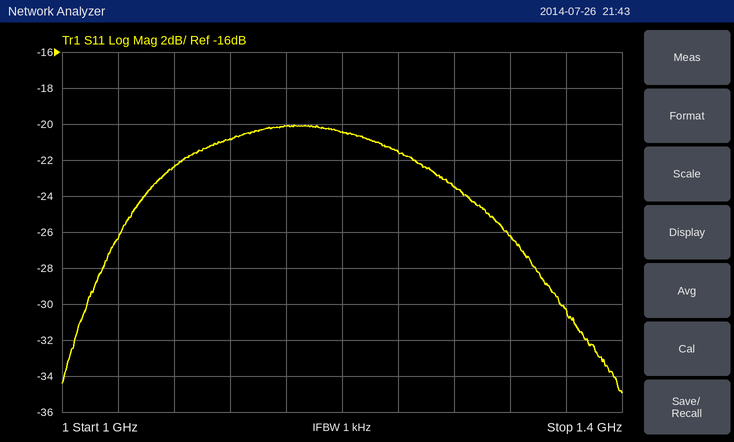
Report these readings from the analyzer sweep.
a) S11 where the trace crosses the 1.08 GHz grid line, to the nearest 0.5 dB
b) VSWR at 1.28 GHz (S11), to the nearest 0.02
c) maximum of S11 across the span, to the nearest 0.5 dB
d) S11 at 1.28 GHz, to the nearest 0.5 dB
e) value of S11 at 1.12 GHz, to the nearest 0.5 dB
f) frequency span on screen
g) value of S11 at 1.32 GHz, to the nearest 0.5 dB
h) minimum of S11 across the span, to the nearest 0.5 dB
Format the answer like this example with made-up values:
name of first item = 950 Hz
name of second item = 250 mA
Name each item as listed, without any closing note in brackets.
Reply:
S11 where the trace crosses the 1.08 GHz grid line, to the nearest 0.5 dB = -22.5 dB
VSWR at 1.28 GHz (S11), to the nearest 0.02 = 1.14
maximum of S11 across the span, to the nearest 0.5 dB = -20.0 dB
S11 at 1.28 GHz, to the nearest 0.5 dB = -23.5 dB
value of S11 at 1.12 GHz, to the nearest 0.5 dB = -21.0 dB
frequency span on screen = 400 MHz
value of S11 at 1.32 GHz, to the nearest 0.5 dB = -26.0 dB
minimum of S11 across the span, to the nearest 0.5 dB = -35.0 dB
